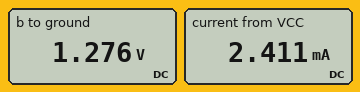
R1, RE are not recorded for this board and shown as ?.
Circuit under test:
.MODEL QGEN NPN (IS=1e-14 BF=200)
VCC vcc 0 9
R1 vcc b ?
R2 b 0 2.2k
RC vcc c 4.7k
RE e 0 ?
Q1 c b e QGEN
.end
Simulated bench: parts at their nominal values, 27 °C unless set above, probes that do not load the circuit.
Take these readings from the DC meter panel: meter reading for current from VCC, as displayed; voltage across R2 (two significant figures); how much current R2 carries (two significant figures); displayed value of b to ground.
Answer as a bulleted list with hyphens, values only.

- 2.411 mA
- 1.3 V
- 580 µA
- 1.276 V
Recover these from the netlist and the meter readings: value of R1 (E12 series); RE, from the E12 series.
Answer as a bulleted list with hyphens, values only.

- 12 kΩ
- 330 Ω
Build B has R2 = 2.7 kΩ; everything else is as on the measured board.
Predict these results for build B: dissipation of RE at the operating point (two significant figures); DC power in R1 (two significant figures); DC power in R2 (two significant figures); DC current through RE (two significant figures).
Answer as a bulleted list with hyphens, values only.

- 1.2 mW
- 4.9 mW
- 630 µW
- 1.9 mA
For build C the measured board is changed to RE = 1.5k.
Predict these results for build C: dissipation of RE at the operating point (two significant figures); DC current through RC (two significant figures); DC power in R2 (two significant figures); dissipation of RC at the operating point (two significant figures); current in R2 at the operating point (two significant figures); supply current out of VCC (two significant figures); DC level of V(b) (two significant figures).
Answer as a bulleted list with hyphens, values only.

- 380 µW
- 500 µA
- 880 µW
- 1.2 mW
- 630 µA
- 1.1 mA
- 1.4 V
